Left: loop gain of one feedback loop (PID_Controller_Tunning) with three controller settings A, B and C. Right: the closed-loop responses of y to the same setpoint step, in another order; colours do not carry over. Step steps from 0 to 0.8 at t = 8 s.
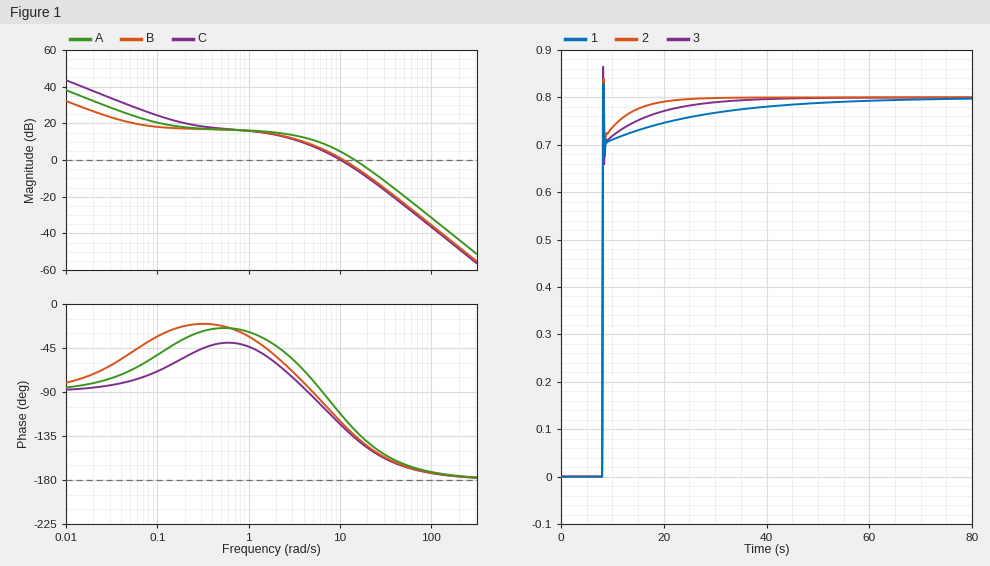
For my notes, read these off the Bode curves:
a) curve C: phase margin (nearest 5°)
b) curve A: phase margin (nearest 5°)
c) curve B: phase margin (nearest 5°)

55°
50°
55°
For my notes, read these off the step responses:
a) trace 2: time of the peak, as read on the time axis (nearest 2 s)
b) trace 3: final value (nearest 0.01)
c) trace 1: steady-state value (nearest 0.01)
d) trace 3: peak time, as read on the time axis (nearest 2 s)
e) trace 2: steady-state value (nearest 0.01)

8 s
0.80
0.80
8 s
0.80
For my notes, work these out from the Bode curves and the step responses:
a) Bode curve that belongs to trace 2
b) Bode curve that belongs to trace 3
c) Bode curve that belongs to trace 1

C
A
B
